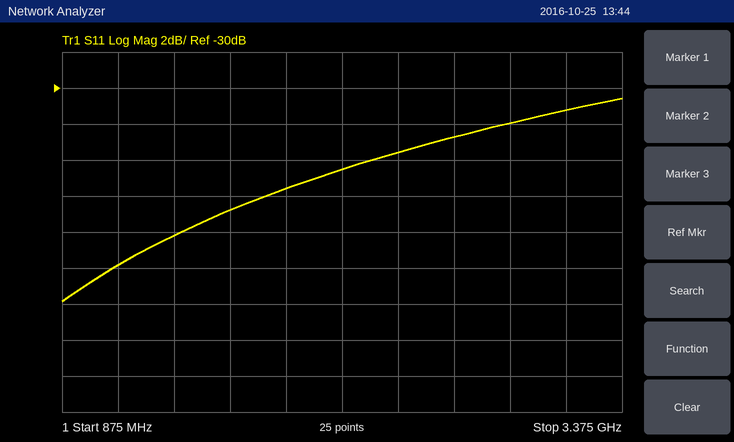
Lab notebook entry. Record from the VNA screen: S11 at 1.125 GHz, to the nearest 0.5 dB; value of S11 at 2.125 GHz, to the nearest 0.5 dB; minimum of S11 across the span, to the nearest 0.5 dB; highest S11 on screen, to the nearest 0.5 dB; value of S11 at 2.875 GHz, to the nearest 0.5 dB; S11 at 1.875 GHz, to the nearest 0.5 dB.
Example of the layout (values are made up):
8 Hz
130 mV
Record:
-40.0 dB
-34.5 dB
-42.0 dB
-30.5 dB
-32.0 dB
-35.5 dB
